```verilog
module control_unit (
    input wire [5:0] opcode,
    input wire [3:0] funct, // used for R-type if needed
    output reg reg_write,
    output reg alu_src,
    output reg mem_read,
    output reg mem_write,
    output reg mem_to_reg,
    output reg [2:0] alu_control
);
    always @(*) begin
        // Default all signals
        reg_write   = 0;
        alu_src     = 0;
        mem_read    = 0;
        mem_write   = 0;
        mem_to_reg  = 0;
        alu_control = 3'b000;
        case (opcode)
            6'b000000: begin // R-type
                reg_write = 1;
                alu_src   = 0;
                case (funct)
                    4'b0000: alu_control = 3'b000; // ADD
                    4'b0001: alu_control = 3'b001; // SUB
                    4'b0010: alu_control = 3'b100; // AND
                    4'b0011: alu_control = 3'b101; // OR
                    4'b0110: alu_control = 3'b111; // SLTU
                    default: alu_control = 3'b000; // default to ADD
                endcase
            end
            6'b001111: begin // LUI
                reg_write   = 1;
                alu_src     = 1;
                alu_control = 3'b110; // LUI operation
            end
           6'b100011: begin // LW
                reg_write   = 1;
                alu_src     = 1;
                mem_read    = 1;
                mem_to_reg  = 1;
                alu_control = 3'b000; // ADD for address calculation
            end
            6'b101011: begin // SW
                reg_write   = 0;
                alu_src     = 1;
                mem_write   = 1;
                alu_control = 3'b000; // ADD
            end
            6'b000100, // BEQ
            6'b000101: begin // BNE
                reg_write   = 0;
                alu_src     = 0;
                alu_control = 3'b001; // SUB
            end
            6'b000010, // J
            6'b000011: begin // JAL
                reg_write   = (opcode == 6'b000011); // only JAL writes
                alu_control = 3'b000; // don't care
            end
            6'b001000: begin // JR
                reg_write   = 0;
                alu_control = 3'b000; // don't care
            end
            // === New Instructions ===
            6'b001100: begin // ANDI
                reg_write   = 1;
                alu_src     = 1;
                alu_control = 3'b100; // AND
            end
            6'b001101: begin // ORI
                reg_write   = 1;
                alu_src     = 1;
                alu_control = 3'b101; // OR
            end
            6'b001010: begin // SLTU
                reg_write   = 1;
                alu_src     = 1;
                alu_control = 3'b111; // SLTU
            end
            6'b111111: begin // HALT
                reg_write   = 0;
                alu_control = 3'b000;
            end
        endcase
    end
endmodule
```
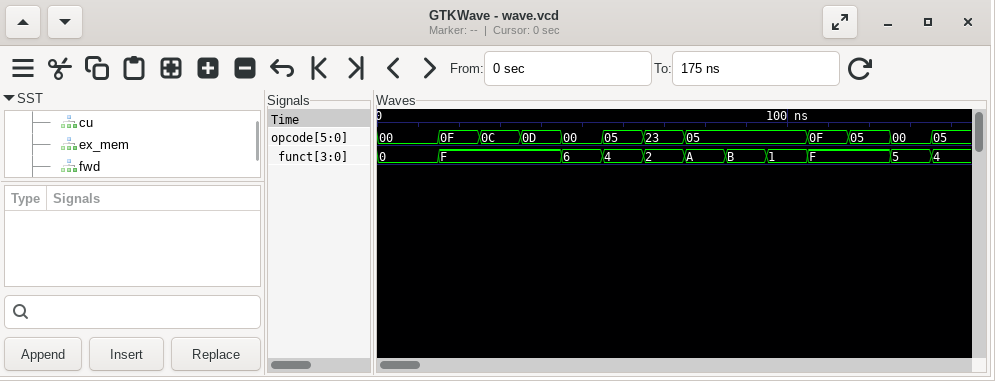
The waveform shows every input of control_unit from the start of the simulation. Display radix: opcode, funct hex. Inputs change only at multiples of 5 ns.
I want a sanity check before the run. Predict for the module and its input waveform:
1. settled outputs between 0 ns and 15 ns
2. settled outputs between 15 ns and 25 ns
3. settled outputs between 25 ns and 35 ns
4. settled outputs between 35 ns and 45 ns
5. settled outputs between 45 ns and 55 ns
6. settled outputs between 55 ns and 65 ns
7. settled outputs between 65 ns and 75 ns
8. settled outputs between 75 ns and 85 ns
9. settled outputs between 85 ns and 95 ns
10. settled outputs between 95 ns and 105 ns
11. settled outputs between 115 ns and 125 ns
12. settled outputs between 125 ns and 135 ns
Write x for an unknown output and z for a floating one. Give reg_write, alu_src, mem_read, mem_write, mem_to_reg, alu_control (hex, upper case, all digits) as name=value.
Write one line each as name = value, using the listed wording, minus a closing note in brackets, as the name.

settled outputs between 0 ns and 15 ns = reg_write=1, alu_src=0, mem_read=0, mem_write=0, mem_to_reg=0, alu_control=0
settled outputs between 15 ns and 25 ns = reg_write=1, alu_src=1, mem_read=0, mem_write=0, mem_to_reg=0, alu_control=6
settled outputs between 25 ns and 35 ns = reg_write=1, alu_src=1, mem_read=0, mem_write=0, mem_to_reg=0, alu_control=4
settled outputs between 35 ns and 45 ns = reg_write=1, alu_src=1, mem_read=0, mem_write=0, mem_to_reg=0, alu_control=5
settled outputs between 45 ns and 55 ns = reg_write=1, alu_src=0, mem_read=0, mem_write=0, mem_to_reg=0, alu_control=7
settled outputs between 55 ns and 65 ns = reg_write=0, alu_src=0, mem_read=0, mem_write=0, mem_to_reg=0, alu_control=1
settled outputs between 65 ns and 75 ns = reg_write=1, alu_src=1, mem_read=1, mem_write=0, mem_to_reg=1, alu_control=0
settled outputs between 75 ns and 85 ns = reg_write=0, alu_src=0, mem_read=0, mem_write=0, mem_to_reg=0, alu_control=1
settled outputs between 85 ns and 95 ns = reg_write=0, alu_src=0, mem_read=0, mem_write=0, mem_to_reg=0, alu_control=1
settled outputs between 95 ns and 105 ns = reg_write=0, alu_src=0, mem_read=0, mem_write=0, mem_to_reg=0, alu_control=1
settled outputs between 115 ns and 125 ns = reg_write=0, alu_src=0, mem_read=0, mem_write=0, mem_to_reg=0, alu_control=1
settled outputs between 125 ns and 135 ns = reg_write=1, alu_src=0, mem_read=0, mem_write=0, mem_to_reg=0, alu_control=0
